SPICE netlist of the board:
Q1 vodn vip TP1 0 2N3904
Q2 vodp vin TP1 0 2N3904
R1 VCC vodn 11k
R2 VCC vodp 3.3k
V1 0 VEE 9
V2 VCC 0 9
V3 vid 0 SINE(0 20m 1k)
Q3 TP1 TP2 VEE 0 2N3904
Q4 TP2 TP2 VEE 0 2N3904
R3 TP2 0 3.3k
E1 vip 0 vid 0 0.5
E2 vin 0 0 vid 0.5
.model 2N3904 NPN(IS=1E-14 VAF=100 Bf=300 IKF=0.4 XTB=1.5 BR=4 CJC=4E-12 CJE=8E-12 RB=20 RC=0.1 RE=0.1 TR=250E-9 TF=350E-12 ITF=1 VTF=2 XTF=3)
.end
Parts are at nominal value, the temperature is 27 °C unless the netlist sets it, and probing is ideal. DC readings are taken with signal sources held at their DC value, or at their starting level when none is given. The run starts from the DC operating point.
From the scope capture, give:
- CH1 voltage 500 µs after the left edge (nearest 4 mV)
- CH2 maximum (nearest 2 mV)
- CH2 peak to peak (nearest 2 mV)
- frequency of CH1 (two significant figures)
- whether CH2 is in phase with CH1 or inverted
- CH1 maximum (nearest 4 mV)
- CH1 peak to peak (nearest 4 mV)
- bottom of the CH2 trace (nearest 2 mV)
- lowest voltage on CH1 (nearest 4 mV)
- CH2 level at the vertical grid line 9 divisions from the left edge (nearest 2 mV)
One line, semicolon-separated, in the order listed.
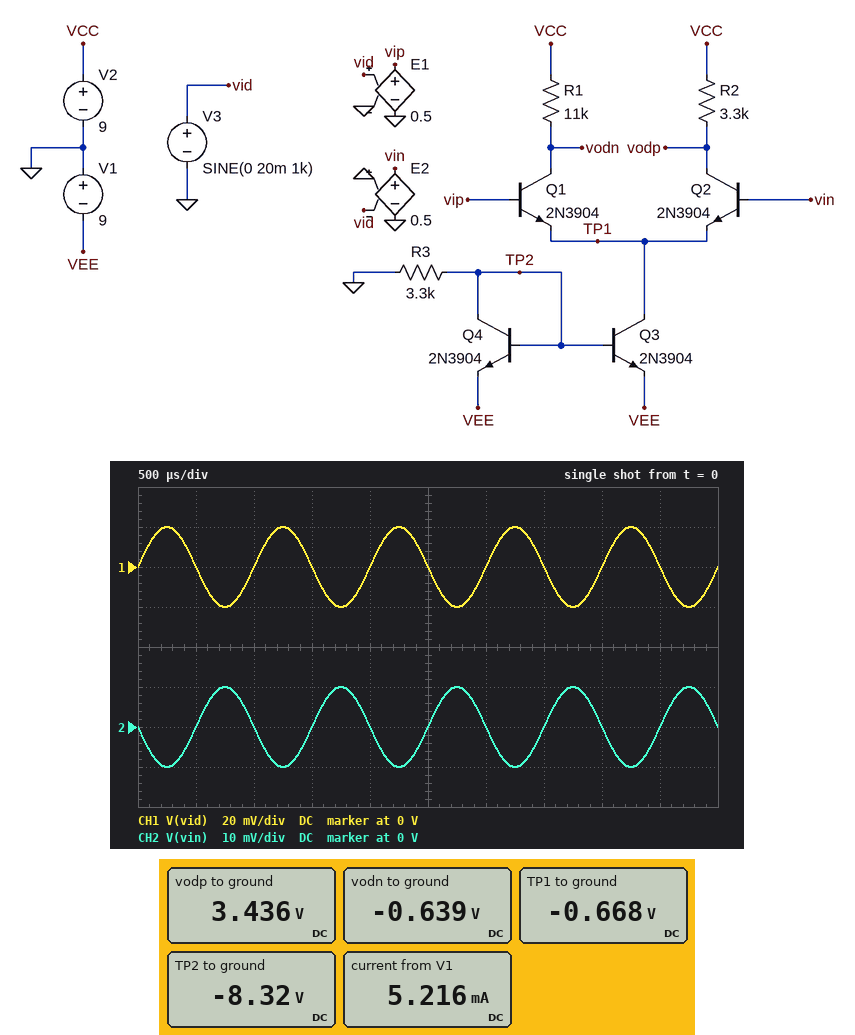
0 V; 10 mV; 20 mV; 1.0 kHz; inverted; 20 mV; 40 mV; -10 mV; -20 mV; 0 V
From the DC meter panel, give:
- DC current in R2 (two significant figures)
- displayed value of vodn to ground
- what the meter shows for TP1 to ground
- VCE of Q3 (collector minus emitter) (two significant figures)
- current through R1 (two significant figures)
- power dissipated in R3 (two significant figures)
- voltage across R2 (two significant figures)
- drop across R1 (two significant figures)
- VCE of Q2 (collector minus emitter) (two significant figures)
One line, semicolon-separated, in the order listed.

1.7 mA; -0.639 V; -0.668 V; 8.3 V; 880 µA; 21 mW; 5.6 V; 9.6 V; 4.1 V
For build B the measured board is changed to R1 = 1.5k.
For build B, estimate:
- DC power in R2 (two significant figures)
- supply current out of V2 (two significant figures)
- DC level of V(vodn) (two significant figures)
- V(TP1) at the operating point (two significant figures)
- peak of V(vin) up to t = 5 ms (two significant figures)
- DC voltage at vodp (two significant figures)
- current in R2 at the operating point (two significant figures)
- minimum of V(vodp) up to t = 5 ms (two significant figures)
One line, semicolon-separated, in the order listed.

5.8 mW; 2.7 mA; 7.0 V; -660 mV; 10 mV; 4.6 V; 1.3 mA; 3.0 V
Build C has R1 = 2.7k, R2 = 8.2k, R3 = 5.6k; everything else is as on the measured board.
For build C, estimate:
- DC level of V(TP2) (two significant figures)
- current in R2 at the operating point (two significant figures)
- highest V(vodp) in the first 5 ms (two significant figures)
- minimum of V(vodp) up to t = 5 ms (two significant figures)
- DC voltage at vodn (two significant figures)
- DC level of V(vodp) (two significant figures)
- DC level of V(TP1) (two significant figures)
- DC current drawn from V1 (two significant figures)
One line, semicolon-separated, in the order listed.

-8.3 V; 780 µA; 4.9 V; 310 mV; 6.8 V; 2.6 V; -650 mV; 3.1 mA
